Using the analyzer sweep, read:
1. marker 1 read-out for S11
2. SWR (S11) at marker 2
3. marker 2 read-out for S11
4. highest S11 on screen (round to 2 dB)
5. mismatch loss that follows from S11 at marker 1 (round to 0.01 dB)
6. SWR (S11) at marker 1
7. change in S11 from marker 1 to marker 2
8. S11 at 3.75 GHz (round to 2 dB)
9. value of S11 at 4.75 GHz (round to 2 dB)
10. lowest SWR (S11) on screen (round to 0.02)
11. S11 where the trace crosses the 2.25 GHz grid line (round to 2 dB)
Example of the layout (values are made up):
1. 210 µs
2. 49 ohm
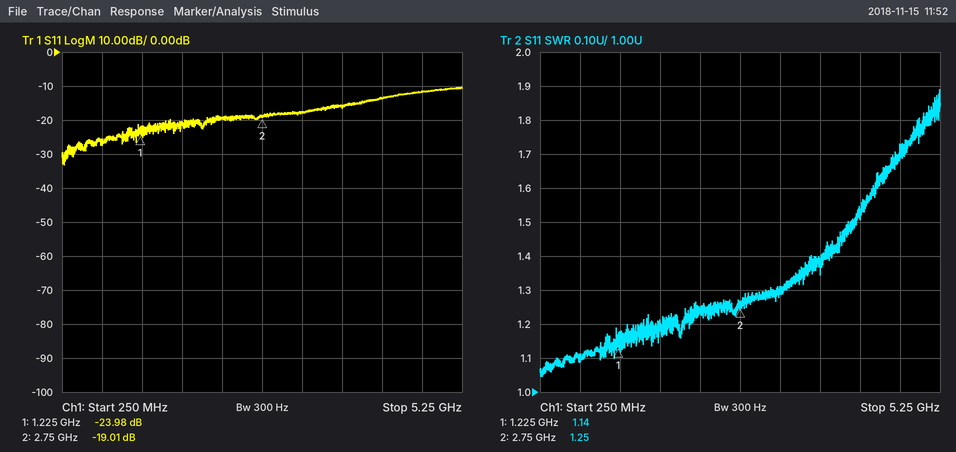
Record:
1. -23.98 dB
2. 1.25
3. -19.01 dB
4. -10 dB
5. 0.02 dB
6. 1.14
7. 4.97 dB
8. -16 dB
9. -12 dB
10. 1.04
11. -20 dB
